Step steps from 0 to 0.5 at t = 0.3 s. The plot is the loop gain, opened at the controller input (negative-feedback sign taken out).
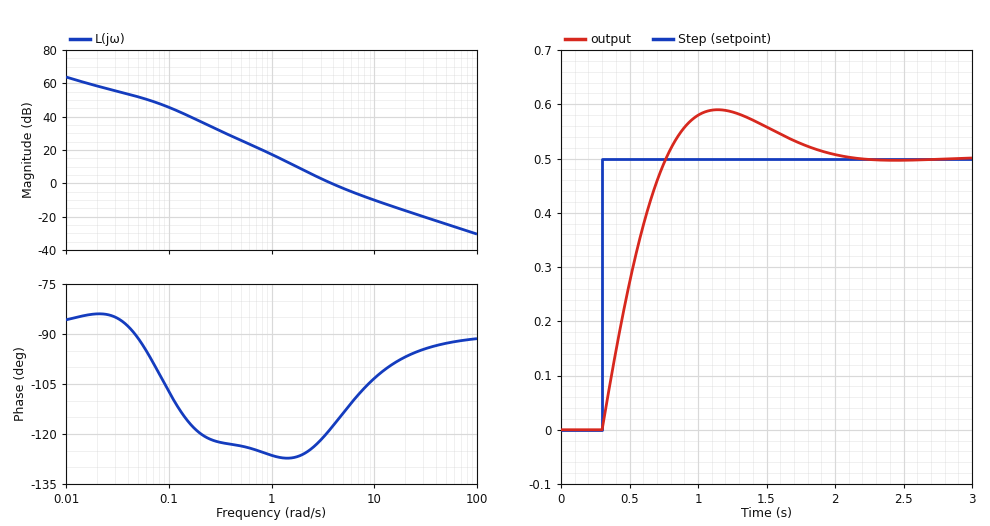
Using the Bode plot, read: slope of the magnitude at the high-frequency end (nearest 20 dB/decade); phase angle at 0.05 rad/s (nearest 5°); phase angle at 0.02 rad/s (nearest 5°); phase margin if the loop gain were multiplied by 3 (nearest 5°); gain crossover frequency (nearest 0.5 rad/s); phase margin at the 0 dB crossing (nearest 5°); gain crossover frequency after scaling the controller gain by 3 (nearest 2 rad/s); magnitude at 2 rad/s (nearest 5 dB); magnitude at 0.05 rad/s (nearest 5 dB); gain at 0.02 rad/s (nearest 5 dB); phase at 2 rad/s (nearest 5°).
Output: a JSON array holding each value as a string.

["-20 dB/decade", "-90°", "-85°", "75°", "4.0 rad/s", "60°", "10 rad/s", "10 dB", "50 dB", "60 dB", "-125°"]
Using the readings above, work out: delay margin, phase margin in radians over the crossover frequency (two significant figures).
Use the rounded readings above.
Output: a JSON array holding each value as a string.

["0.26 s"]
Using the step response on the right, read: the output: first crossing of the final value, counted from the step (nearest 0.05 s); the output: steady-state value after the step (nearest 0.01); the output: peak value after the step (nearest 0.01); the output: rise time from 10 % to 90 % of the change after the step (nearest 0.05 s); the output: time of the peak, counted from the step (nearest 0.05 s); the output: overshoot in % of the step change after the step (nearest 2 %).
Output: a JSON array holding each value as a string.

["0.45 s", "0.50", "0.59", "0.35 s", "0.85 s", "18 %"]
